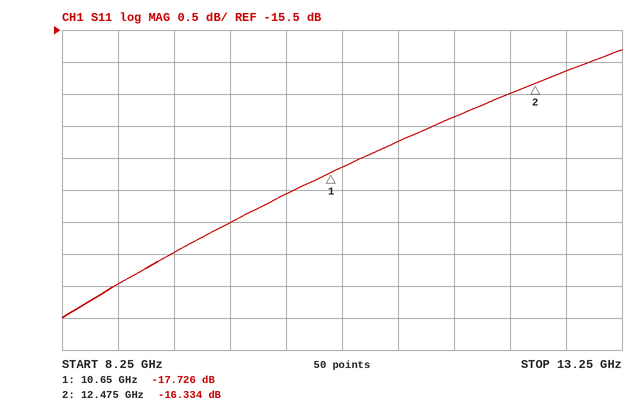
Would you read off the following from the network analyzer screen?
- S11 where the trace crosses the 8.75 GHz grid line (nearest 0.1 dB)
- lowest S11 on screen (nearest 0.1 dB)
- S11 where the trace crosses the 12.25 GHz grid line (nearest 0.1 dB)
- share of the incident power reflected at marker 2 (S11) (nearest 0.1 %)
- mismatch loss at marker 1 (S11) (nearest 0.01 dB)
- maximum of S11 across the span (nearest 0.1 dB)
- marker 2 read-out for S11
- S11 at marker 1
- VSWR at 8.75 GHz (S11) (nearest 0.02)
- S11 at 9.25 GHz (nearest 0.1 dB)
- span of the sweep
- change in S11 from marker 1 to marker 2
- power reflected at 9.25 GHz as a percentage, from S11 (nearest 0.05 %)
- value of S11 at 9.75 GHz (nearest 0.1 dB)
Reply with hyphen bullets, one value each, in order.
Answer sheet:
- -19.5 dB
- -20.0 dB
- -16.5 dB
- 2.3 %
- 0.07 dB
- -15.8 dB
- -16.334 dB
- -17.726 dB
- 1.24
- -19.0 dB
- 5 GHz
- 1.392 dB
- 1.25 %
- -18.5 dB
